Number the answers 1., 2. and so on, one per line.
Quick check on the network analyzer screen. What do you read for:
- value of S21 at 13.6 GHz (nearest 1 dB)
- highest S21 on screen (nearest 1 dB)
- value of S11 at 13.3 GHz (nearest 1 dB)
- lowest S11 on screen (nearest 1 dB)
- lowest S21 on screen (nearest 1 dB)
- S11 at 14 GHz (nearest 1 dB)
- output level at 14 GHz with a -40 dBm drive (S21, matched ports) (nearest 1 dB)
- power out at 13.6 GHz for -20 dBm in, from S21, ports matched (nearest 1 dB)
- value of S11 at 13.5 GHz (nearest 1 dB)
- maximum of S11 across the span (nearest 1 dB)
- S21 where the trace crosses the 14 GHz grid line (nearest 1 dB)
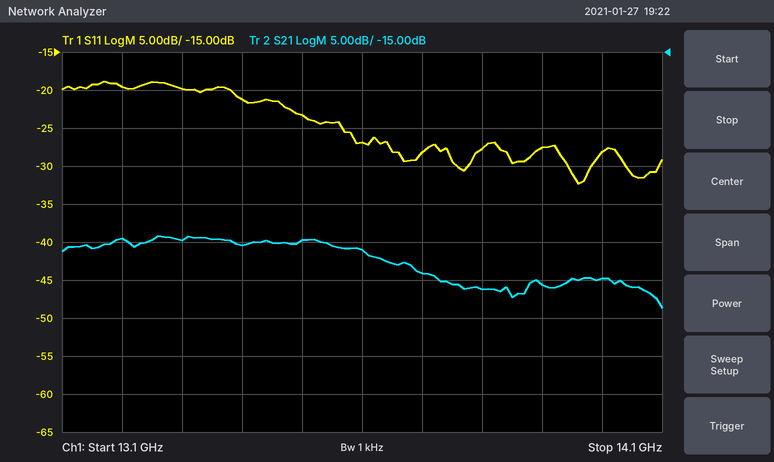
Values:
1. -41 dB
2. -39 dB
3. -20 dB
4. -32 dB
5. -49 dB
6. -28 dB
7. -85 dBm
8. -61 dBm
9. -23 dB
10. -19 dB
11. -45 dB
